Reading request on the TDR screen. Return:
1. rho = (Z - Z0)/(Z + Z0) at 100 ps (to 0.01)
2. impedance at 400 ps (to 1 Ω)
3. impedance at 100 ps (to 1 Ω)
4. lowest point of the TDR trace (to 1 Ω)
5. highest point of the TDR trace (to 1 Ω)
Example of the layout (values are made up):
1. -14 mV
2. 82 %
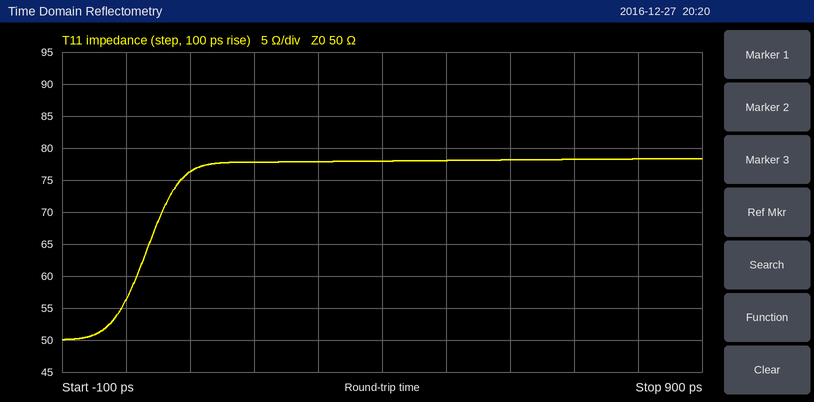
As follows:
1. +0.21
2. 78 Ω
3. 76 Ω
4. 50 Ω
5. 78 Ω
